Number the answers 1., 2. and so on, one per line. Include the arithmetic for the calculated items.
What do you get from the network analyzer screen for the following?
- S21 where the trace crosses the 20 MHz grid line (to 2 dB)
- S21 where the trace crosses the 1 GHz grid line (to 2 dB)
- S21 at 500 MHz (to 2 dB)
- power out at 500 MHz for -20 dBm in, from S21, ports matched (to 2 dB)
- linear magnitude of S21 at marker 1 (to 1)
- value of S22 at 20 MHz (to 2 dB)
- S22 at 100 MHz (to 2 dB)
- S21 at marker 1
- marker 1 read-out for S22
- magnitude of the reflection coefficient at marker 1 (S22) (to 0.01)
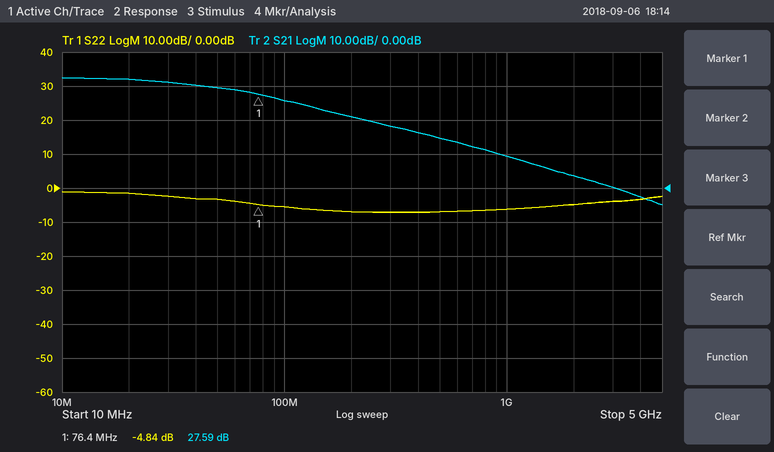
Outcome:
1. 32 dB
2. 10 dB
3. 14 dB
4. -20 dBm + (14 dB) = -6 dBm
5. 10^(27.59/20) ≈ 24
6. -2 dB
7. -6 dB
8. 27.59 dB
9. -4.84 dB
10. 10^(-4.84/20) ≈ 0.57
